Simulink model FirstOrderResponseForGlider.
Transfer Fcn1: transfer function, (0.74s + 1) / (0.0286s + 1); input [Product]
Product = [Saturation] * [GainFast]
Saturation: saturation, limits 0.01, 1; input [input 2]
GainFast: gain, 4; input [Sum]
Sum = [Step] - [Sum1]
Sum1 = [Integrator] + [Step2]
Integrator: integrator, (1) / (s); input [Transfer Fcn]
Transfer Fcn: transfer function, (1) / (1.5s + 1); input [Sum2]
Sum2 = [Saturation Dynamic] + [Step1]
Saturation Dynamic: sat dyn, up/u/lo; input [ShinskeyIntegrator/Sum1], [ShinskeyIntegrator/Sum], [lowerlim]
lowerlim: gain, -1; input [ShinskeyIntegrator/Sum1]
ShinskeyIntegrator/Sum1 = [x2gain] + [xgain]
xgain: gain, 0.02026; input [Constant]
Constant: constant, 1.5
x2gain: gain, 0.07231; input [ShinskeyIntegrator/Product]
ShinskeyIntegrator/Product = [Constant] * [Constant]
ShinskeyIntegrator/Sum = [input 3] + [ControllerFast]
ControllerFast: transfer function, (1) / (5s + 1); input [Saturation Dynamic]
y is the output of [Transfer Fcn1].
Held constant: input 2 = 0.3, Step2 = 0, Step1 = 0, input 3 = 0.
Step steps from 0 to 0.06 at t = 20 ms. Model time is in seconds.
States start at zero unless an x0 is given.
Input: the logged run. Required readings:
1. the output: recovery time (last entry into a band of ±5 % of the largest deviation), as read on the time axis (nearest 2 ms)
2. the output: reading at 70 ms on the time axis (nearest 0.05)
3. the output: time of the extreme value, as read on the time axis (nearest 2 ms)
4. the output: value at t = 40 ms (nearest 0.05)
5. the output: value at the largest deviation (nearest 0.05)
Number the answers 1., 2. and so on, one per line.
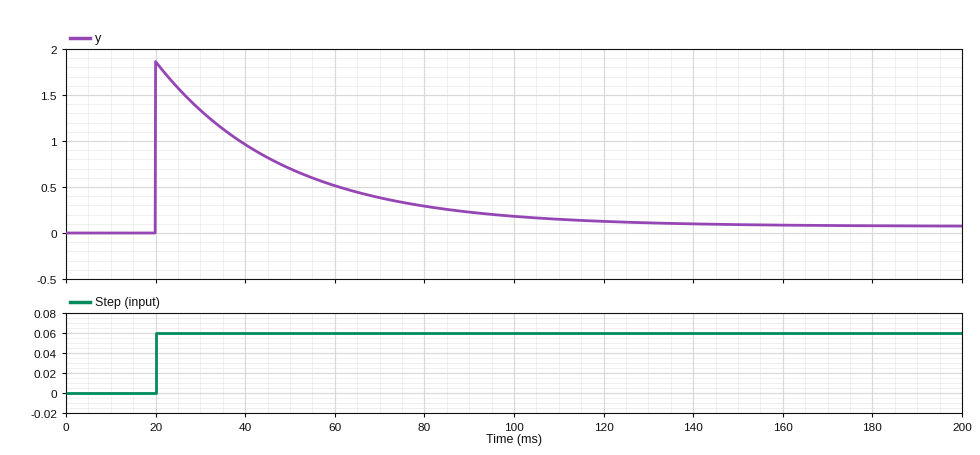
1. 104 ms
2. 0.40
3. 20 ms
4. 0.95
5. 1.85
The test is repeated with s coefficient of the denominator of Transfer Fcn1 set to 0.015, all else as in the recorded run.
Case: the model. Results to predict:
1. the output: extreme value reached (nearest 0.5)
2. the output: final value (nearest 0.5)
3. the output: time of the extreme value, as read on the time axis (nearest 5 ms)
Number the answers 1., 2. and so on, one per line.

1. 3.5
2. 0.0
3. 20 ms
